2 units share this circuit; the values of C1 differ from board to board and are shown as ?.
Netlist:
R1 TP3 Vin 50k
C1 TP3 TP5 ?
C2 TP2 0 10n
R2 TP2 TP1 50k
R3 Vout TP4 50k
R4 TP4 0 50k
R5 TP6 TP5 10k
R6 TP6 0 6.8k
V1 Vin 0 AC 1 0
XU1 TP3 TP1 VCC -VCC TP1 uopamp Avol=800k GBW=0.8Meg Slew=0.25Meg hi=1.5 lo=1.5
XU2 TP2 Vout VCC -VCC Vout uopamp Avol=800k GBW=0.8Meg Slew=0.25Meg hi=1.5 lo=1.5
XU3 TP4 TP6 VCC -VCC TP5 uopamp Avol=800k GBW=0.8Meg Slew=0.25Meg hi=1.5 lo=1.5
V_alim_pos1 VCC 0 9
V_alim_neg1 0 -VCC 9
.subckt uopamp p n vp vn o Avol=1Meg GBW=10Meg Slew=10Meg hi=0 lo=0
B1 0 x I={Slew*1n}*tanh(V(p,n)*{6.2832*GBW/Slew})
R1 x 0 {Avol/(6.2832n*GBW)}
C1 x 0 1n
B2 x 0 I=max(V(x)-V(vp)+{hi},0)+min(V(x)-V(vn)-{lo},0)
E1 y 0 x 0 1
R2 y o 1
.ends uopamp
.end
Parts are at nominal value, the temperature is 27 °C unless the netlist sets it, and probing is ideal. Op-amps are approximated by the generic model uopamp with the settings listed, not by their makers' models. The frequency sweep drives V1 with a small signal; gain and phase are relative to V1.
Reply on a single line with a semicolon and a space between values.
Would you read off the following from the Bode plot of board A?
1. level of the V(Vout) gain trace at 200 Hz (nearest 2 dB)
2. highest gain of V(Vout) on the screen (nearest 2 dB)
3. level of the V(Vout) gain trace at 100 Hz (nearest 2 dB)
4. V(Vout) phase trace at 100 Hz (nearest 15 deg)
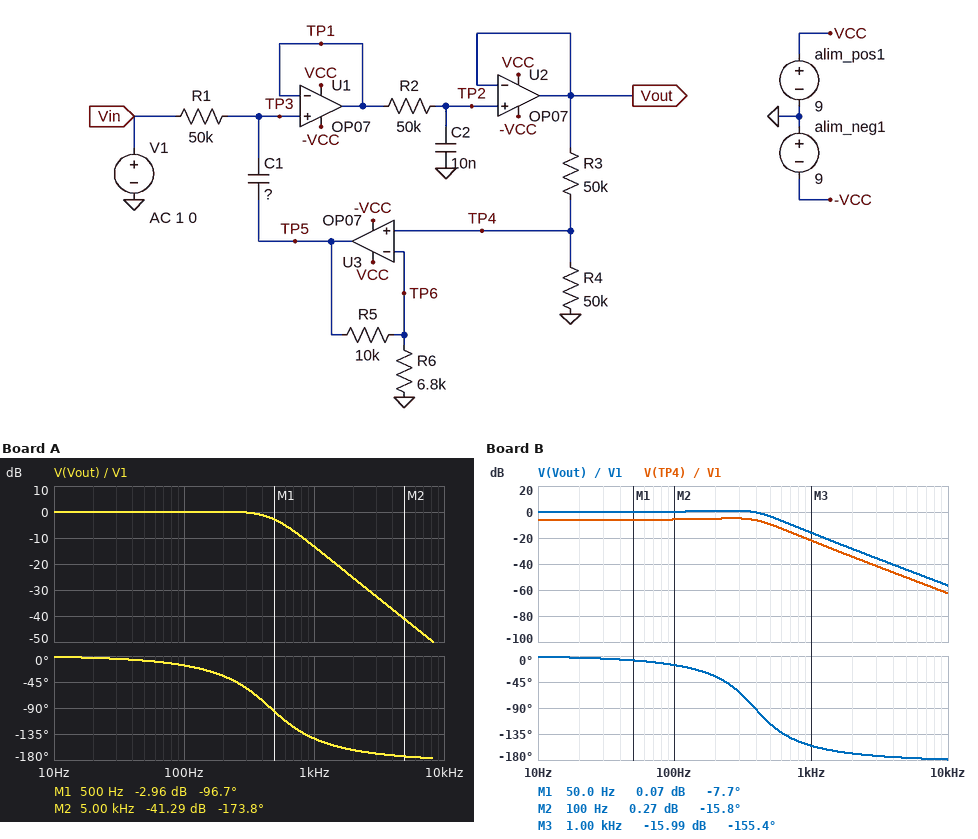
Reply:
0 dB; 0 dB; 0 dB; -15 deg
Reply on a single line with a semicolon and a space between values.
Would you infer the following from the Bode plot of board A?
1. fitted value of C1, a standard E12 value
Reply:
4.7 nF
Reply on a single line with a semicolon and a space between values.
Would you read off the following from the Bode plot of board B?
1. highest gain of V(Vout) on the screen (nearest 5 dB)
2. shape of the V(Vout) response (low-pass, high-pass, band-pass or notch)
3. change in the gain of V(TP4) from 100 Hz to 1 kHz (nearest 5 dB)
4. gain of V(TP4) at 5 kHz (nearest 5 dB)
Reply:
0 dB; low-pass; -15 dB; -50 dB
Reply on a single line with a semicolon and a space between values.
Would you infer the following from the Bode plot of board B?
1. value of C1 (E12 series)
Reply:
6.8 nF
